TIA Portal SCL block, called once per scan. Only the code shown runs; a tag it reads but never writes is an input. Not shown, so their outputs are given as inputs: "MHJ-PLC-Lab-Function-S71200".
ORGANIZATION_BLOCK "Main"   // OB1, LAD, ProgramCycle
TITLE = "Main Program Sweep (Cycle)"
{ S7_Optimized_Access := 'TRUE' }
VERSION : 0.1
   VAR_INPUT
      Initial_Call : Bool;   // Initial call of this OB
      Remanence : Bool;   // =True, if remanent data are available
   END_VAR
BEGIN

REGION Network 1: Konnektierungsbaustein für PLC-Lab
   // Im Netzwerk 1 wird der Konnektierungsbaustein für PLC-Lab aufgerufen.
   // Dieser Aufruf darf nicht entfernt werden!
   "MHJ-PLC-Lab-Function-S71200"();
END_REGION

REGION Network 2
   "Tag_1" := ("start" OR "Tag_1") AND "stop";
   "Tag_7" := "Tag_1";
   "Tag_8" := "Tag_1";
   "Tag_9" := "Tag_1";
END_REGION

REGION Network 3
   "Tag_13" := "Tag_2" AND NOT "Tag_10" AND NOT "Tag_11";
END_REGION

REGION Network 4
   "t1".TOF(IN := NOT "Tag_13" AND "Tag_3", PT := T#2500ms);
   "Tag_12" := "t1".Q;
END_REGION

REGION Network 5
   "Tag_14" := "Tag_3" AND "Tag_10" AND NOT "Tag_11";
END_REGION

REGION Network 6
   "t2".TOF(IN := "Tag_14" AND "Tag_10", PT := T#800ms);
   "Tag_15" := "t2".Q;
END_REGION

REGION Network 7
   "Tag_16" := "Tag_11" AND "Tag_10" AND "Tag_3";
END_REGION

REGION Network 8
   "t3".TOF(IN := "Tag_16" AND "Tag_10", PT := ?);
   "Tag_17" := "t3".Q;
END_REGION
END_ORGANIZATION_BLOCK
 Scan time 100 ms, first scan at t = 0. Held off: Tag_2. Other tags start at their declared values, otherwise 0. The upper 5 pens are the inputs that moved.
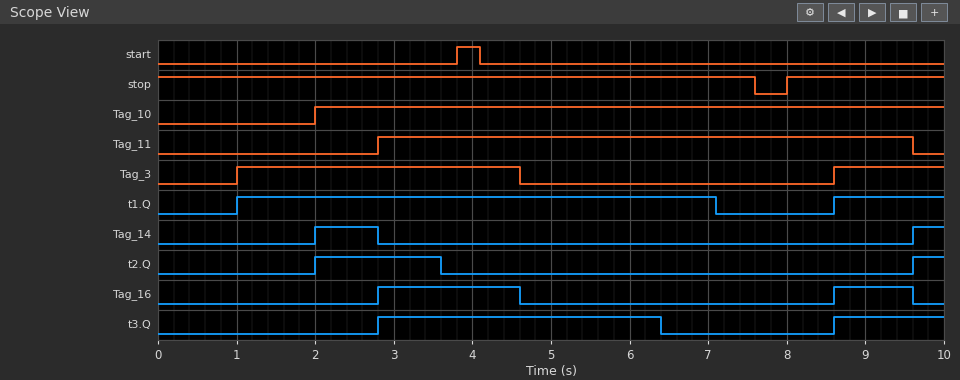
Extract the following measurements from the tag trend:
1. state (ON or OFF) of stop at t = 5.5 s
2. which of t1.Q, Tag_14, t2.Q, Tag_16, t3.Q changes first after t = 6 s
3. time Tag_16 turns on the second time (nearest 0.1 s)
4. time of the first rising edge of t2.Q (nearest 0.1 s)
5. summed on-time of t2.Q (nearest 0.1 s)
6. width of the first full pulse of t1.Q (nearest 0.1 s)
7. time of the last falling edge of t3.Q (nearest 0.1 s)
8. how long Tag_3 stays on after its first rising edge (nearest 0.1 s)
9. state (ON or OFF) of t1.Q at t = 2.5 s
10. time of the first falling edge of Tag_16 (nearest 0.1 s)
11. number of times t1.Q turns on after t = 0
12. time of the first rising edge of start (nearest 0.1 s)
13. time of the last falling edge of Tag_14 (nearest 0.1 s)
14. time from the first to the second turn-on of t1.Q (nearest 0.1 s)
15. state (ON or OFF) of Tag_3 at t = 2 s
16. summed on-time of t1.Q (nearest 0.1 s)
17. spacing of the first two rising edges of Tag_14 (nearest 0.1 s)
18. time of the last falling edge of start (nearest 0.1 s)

ON
t3.Q
8.6 s
2.0 s
2.0 s
6.1 s
6.4 s
3.6 s
ON
4.6 s
2
3.8 s
2.8 s
7.6 s
ON
7.5 s
7.6 s
4.1 s
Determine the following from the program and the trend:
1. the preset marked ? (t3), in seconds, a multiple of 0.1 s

1.8 s
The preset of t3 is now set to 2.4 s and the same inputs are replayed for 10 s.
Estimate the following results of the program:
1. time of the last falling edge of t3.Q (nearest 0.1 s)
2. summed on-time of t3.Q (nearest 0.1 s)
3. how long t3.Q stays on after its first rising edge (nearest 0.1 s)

7.0 s
5.6 s
4.2 s
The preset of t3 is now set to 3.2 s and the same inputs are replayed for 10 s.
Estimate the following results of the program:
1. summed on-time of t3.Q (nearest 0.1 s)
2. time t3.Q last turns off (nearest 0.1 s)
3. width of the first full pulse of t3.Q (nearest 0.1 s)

6.4 s
7.8 s
5.0 s
